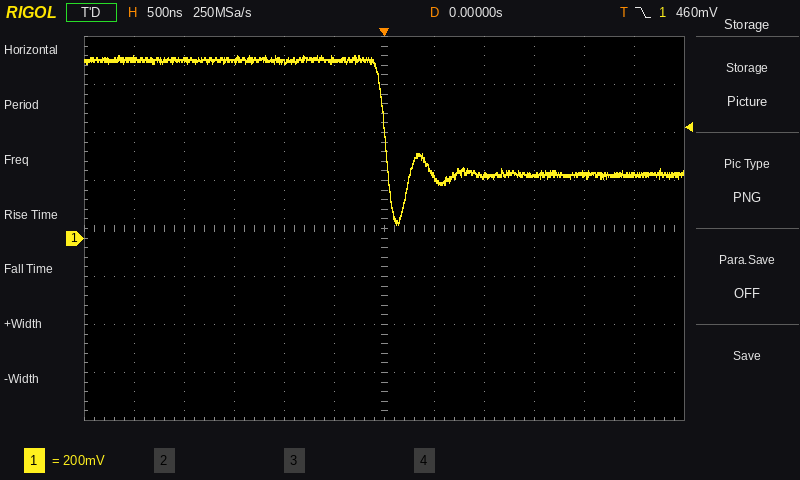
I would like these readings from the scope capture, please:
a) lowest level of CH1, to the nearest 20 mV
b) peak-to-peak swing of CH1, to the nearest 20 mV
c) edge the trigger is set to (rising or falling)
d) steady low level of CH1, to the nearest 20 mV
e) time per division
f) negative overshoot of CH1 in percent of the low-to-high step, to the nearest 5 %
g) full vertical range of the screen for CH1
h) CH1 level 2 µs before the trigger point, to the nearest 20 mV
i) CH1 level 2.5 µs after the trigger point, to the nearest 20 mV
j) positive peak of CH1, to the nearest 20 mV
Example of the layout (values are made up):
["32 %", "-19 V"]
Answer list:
["60 mV", "700 mV", "falling", "260 mV", "500 ns", "45 %", "1.6 V", "740 mV", "260 mV", "760 mV"]
